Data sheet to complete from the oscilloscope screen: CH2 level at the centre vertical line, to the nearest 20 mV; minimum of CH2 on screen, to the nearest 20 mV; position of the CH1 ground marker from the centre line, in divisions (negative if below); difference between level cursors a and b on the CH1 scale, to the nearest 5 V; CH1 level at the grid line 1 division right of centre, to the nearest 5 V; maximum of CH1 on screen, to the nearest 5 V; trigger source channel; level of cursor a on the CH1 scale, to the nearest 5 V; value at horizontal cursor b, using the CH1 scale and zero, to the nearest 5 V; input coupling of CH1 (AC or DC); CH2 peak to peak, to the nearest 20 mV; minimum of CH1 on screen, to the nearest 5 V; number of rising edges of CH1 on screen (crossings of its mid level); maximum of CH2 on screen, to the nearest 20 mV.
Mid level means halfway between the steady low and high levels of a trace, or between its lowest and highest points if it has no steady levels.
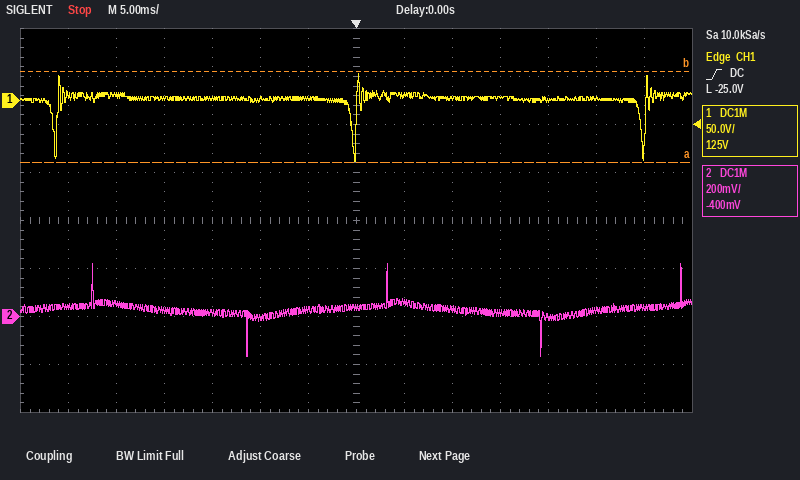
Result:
40 mV
-160 mV
+2.5 div
95 V
5 V
30 V
CH1
-65 V
30 V
DC
380 mV
-65 V
3
220 mV
